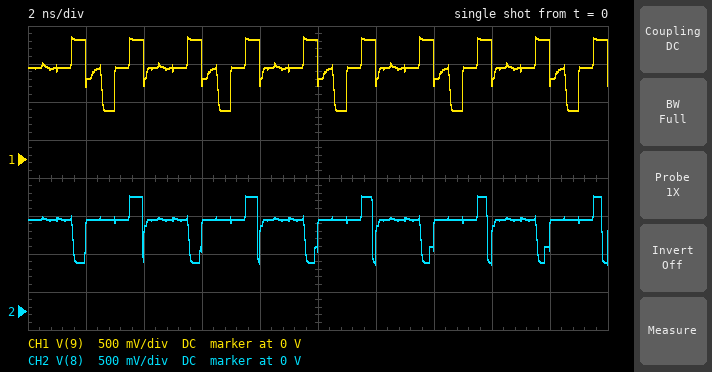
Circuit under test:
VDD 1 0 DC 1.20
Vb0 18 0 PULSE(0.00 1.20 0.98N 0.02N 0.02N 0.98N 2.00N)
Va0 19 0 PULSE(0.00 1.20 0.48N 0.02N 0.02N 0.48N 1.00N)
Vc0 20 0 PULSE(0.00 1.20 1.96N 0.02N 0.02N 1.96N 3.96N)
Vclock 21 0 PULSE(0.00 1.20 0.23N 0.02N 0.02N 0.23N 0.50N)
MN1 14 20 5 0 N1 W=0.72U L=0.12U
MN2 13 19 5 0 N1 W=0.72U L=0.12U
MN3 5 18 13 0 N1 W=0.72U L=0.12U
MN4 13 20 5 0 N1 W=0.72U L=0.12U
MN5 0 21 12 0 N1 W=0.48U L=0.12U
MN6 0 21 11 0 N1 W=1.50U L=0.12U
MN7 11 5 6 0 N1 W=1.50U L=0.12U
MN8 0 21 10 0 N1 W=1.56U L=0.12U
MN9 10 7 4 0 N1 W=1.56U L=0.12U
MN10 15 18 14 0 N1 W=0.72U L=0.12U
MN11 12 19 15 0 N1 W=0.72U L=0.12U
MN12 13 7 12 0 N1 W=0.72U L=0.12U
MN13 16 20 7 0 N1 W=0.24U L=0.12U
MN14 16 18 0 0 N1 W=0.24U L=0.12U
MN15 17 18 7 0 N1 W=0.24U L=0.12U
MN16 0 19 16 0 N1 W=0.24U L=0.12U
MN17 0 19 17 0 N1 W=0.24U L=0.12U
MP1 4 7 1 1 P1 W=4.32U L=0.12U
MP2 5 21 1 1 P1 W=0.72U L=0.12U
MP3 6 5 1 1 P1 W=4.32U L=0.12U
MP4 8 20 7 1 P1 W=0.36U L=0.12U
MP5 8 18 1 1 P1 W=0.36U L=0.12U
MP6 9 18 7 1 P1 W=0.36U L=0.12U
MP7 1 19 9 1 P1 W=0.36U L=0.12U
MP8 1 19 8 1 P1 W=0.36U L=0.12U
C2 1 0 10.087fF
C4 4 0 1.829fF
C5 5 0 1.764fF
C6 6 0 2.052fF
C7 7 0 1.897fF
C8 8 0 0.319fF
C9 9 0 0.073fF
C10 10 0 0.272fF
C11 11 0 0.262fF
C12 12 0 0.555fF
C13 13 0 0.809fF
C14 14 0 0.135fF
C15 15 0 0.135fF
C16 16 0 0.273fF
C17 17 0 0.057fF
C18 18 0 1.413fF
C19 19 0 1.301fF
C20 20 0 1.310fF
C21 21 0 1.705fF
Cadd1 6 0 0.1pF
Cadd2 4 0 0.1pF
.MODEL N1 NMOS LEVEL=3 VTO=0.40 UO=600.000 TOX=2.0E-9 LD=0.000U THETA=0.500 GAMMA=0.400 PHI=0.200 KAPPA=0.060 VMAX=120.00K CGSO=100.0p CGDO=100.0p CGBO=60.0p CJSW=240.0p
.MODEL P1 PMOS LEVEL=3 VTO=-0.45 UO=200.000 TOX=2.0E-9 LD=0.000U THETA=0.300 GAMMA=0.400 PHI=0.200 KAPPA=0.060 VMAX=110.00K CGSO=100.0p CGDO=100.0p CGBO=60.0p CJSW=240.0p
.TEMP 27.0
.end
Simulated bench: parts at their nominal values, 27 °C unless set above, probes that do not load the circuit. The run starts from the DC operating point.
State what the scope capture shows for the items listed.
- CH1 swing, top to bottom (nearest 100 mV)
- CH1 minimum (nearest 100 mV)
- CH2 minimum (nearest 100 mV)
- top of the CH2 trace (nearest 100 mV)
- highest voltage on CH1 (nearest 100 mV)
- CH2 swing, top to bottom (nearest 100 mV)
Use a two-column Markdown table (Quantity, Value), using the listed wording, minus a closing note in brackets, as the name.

| Quantity | Value |
|---|---|
| CH1 swing, top to bottom | 1.0 V |
| CH1 minimum | 600 mV |
| CH2 minimum | 600 mV |
| top of the CH2 trace | 1.5 V |
| highest voltage on CH1 | 1.6 V |
| CH2 swing, top to bottom | 900 mV |
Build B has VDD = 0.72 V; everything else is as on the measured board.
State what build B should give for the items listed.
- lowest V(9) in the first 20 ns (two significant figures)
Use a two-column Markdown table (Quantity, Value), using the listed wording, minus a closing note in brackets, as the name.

| Quantity | Value |
|---|---|
| lowest V(9) in the first 20 ns | 520 mV |
